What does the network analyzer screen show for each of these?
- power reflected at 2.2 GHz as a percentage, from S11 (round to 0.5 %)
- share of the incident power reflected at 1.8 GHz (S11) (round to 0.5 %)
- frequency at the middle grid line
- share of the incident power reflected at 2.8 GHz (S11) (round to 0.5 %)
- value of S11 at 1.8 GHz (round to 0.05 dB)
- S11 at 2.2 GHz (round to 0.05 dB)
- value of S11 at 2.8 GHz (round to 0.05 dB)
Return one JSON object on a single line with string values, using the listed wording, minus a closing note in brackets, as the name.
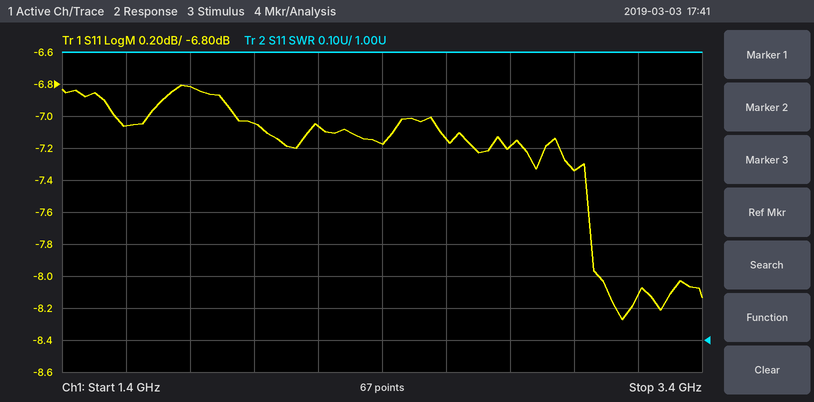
{"power reflected at 2.2 GHz as a percentage, from S11": "19.5 %", "share of the incident power reflected at 1.8 GHz (S11)": "21.0 %", "frequency at the middle grid line": "2.4 GHz", "share of the incident power reflected at 2.8 GHz (S11)": "19.0 %", "value of S11 at 1.8 GHz": "-6.80 dB", "S11 at 2.2 GHz": "-7.05 dB", "value of S11 at 2.8 GHz": "-7.20 dB"}
